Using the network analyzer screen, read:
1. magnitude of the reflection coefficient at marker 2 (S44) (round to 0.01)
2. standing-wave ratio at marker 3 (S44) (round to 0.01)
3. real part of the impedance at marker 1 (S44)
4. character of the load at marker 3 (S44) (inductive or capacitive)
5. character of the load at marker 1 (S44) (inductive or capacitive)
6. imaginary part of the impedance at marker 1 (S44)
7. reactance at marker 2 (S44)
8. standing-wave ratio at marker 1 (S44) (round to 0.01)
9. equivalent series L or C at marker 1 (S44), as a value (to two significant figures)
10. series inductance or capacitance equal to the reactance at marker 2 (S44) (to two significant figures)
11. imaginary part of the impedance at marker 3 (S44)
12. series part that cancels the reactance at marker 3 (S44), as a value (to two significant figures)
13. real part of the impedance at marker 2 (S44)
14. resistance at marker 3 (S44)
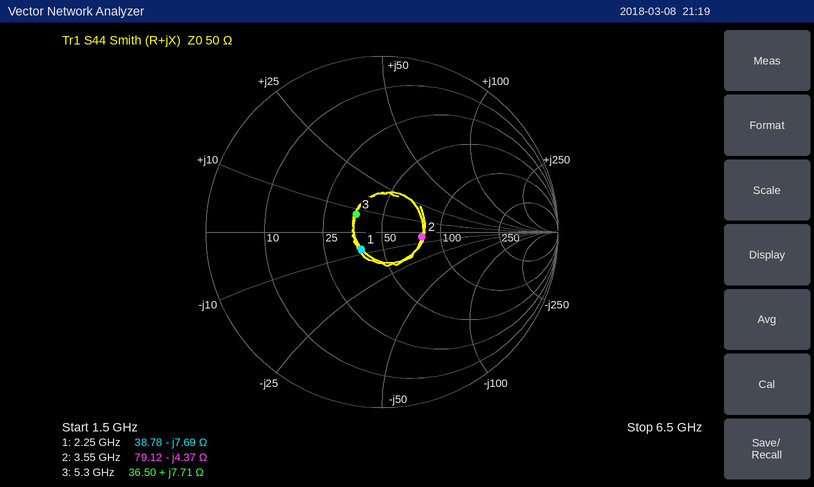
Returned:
0.23
1.44
38.78 Ω
inductive
capacitive
-7.69 Ω
-4.37 Ω
1.36
9.2 pF
10 pF
+7.71 Ω
3.9 pF
79.12 Ω
36.50 Ω
